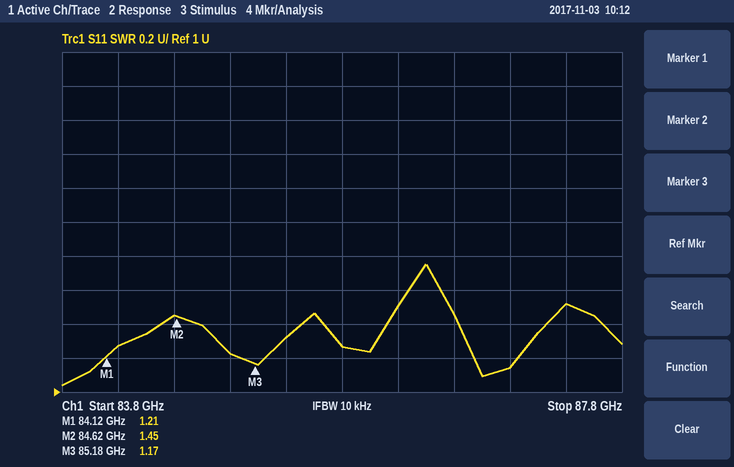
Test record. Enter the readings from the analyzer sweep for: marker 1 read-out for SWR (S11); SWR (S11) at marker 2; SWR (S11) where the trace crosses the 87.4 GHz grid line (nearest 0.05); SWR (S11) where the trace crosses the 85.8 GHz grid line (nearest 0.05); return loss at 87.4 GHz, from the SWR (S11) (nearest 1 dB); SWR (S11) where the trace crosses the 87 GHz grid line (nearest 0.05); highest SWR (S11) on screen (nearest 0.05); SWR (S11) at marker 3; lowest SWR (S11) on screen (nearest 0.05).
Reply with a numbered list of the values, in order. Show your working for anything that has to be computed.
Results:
1. 1.21
2. 1.45
3. 1.50
4. 1.25
5. −20 log10((1.5 − 1)/(1.5 + 1)) ≈ 14 dB
6. 1.15
7. 1.75
8. 1.17
9. 1.05
